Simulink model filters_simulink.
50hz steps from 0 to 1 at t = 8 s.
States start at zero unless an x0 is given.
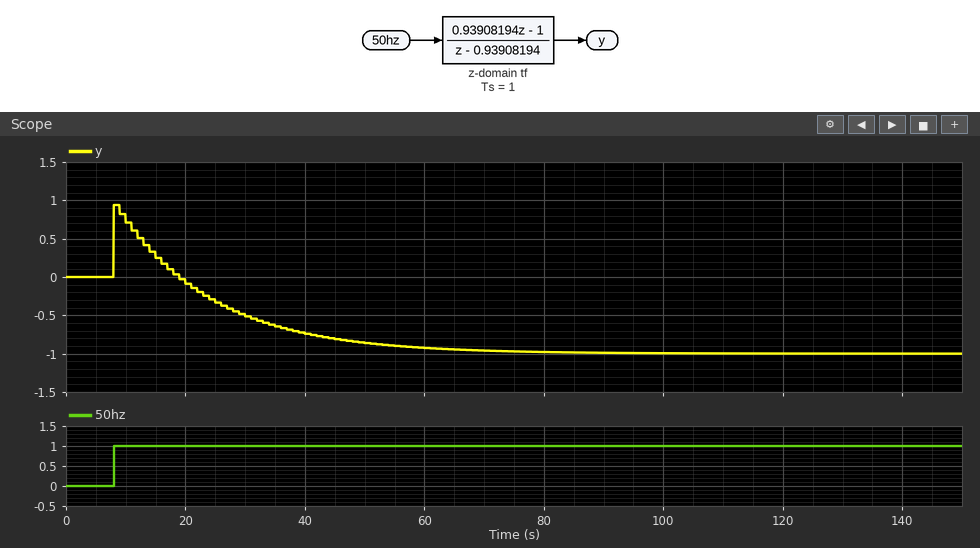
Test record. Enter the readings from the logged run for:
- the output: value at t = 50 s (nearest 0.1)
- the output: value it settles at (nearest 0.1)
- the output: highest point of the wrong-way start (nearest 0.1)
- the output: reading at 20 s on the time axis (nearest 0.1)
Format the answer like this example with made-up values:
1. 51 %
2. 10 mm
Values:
1. -0.9
2. -1.0
3. 0.9
4. -0.1
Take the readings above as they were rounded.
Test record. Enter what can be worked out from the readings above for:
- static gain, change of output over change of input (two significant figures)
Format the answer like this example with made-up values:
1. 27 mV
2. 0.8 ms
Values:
1. -1.0
